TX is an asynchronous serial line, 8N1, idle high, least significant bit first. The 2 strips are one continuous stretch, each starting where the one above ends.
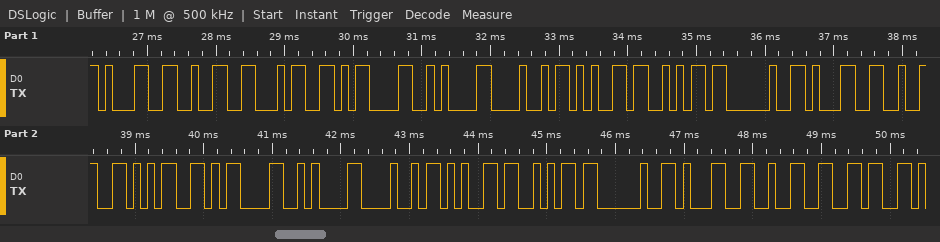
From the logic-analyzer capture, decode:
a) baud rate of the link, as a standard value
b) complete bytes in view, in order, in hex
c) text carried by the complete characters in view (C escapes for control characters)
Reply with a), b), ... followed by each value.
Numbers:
a) 9600 baud
b) 31 32 34 0D 0A 48 65 6A 20 31 32 35 0D 0A 48 65 6A 20 31 32 36
c) "124\r\nHej 125\r\nHej 126"
